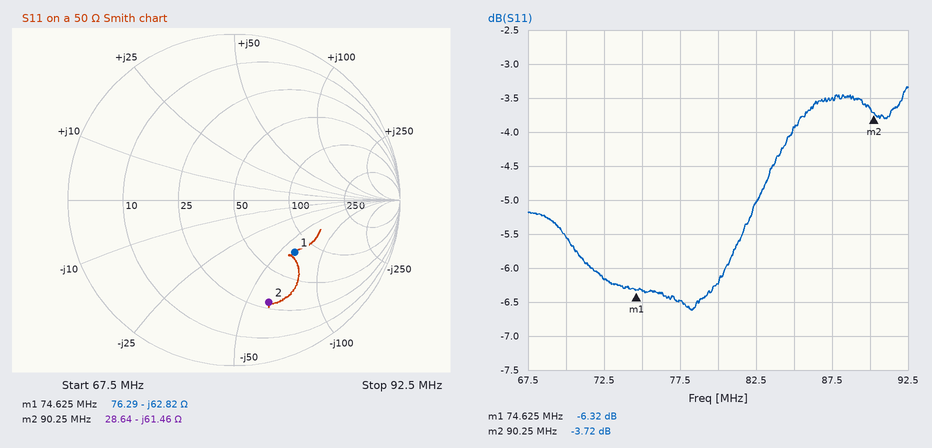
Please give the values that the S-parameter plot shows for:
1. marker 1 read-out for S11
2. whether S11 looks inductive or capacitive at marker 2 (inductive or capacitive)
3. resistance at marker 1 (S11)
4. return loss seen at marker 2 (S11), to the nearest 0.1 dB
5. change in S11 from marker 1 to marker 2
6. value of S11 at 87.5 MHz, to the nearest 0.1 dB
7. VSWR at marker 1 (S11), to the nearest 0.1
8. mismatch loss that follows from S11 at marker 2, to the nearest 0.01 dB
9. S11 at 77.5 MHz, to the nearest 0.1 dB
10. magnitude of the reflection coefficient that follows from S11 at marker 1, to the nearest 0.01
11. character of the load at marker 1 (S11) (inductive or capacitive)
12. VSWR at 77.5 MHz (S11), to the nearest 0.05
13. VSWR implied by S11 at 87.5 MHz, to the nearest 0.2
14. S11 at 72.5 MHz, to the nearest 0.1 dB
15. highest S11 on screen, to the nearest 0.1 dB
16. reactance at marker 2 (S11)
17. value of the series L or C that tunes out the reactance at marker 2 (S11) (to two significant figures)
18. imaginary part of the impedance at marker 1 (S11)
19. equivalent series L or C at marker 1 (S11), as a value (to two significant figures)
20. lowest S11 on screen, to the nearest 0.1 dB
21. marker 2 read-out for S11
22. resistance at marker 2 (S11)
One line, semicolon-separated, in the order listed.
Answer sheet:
-6.32 dB; capacitive; 76.29 Ω; 3.7 dB; 2.60 dB; -3.5 dB; 2.9; 2.40 dB; -6.5 dB; 0.48; capacitive; 2.80; 5.0; -6.2 dB; -3.3 dB; -61.46 Ω; 110 nH; -62.82 Ω; 34 pF; -6.6 dB; -3.72 dB; 28.64 Ω
